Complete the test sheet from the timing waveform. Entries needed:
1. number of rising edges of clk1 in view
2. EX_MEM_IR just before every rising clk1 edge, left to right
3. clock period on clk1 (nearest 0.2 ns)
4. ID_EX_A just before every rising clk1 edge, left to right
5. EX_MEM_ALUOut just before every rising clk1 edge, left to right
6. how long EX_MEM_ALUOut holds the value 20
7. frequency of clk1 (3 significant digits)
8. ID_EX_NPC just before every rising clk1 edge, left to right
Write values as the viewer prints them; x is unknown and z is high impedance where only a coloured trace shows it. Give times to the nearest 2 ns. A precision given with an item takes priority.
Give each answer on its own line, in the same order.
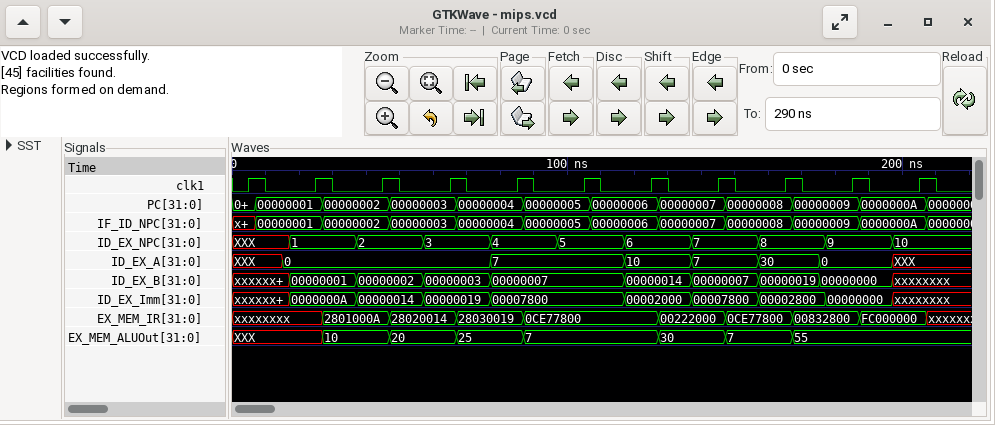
11
xxxxxxxx, xxxxxxxx, 2801000A, 28020014, 28030019, 0CE77800, 0CE77800, 00222000, 0CE77800, 00832800, FC000000
20 ns
XXX, 0, 0, 0, 7, 7, 10, 7, 30, 0, XXX
XXX, XXX, 10, 20, 25, 7, 7, 30, 7, 55, 55
20 ns
50.0 MHz
XXX, 1, 2, 3, 4, 5, 6, 7, 8, 9, 10
